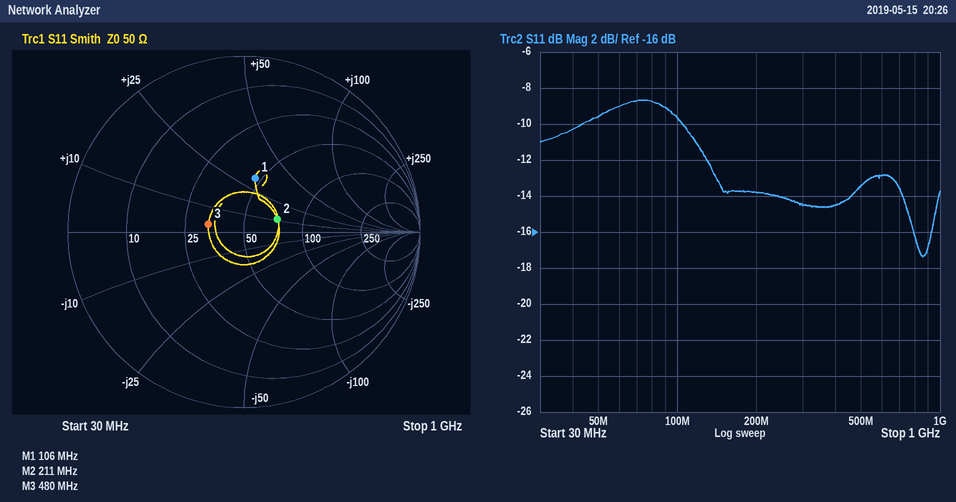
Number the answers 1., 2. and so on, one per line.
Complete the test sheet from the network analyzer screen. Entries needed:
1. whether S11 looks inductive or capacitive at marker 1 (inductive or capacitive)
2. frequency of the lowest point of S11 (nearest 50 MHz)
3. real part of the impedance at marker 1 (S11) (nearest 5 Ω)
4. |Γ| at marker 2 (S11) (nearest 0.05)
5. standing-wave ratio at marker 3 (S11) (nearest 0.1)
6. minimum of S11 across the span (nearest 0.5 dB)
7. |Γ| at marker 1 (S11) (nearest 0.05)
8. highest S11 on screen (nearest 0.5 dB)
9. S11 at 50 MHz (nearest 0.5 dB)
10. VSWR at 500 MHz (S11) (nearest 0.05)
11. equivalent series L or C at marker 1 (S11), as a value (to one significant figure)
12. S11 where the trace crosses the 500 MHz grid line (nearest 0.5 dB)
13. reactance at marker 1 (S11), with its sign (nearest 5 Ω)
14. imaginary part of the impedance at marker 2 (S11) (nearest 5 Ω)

1. inductive
2. 850 MHz
3. 45 Ω
4. 0.20
5. 1.5
6. -17.5 dB
7. 0.30
8. -8.5 dB
9. -9.5 dB
10. 1.55
11. 50 nH
12. -13.5 dB
13. +30 Ω
14. +10 Ω
